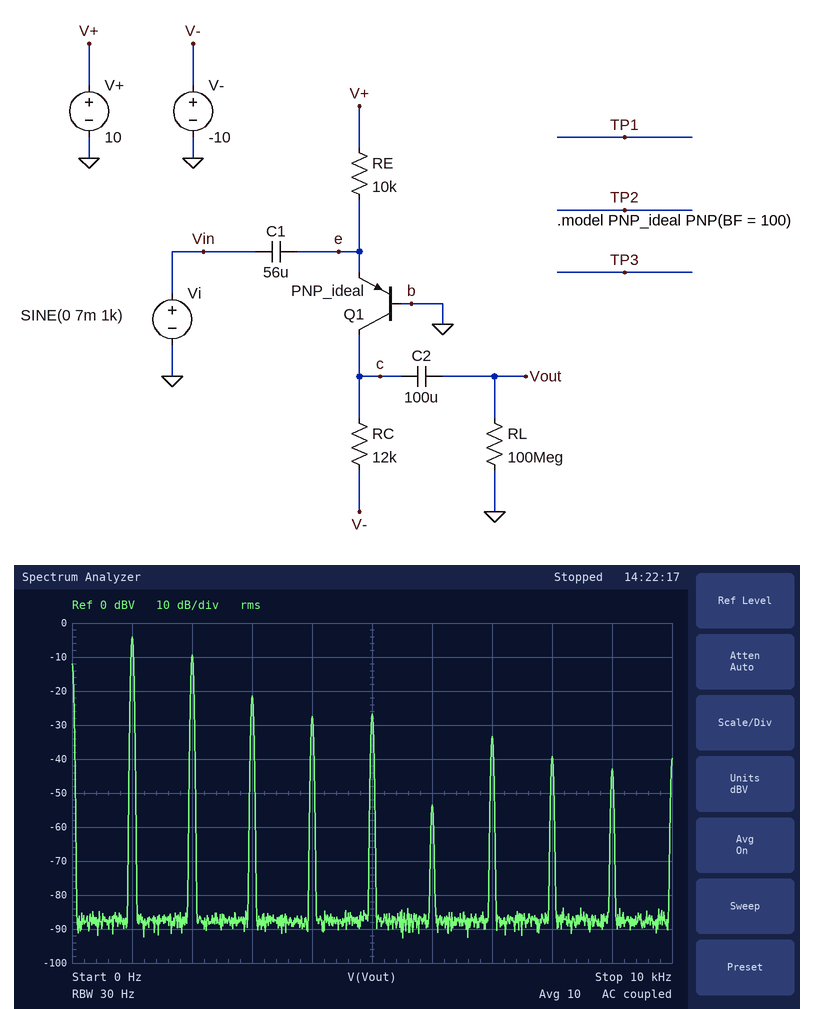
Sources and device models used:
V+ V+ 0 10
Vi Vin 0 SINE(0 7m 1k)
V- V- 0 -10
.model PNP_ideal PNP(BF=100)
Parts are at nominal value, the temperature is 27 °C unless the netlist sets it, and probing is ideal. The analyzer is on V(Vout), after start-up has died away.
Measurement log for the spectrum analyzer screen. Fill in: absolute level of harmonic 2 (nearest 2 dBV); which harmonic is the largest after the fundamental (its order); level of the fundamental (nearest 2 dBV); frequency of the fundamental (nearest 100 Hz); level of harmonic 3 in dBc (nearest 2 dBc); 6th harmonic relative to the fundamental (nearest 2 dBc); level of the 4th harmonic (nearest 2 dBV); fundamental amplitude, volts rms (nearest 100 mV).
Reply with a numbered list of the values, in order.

1. -10 dBV
2. 2
3. -4 dBV
4. 1.0 kHz
5. -18 dBc
6. -50 dBc
7. -28 dBV
8. 600 mV
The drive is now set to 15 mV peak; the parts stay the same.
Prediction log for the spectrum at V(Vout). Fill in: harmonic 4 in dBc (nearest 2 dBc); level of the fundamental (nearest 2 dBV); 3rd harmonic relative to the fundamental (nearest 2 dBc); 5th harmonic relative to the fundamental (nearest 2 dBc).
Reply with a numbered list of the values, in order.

1. -20 dBc
2. 4 dBV
3. -34 dBc
4. -30 dBc
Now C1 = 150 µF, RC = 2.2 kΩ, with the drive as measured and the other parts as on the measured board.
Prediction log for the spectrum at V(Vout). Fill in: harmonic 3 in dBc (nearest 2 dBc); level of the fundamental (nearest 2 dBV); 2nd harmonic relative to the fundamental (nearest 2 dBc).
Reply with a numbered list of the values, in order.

1. -50 dBc
2. -8 dBV
3. -24 dBc
